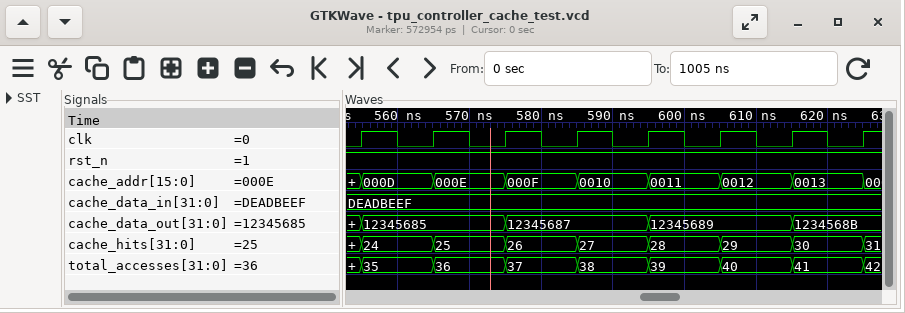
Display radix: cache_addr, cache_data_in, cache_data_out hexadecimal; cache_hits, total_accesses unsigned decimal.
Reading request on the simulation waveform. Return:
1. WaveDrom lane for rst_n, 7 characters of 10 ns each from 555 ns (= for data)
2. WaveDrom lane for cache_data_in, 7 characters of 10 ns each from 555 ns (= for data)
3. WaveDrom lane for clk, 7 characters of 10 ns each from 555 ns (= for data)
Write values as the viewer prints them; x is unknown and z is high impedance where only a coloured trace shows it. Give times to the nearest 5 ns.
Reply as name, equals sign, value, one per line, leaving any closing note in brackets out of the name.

WaveDrom lane for rst_n, 7 characters of 10 ns each from 555 ns = {name: 'rst_n', wave: '1......'}
WaveDrom lane for cache_data_in, 7 characters of 10 ns each from 555 ns = {name: 'cache_data_in', wave: '=......', data: 'DEADBEEF'}
WaveDrom lane for clk, 7 characters of 10 ns each from 555 ns = {name: 'clk', wave: 'p......'}
